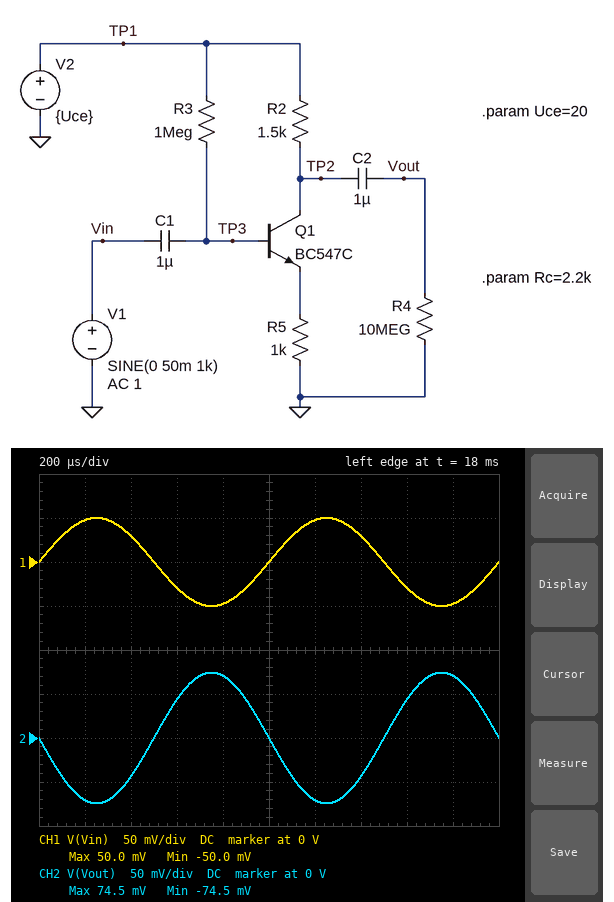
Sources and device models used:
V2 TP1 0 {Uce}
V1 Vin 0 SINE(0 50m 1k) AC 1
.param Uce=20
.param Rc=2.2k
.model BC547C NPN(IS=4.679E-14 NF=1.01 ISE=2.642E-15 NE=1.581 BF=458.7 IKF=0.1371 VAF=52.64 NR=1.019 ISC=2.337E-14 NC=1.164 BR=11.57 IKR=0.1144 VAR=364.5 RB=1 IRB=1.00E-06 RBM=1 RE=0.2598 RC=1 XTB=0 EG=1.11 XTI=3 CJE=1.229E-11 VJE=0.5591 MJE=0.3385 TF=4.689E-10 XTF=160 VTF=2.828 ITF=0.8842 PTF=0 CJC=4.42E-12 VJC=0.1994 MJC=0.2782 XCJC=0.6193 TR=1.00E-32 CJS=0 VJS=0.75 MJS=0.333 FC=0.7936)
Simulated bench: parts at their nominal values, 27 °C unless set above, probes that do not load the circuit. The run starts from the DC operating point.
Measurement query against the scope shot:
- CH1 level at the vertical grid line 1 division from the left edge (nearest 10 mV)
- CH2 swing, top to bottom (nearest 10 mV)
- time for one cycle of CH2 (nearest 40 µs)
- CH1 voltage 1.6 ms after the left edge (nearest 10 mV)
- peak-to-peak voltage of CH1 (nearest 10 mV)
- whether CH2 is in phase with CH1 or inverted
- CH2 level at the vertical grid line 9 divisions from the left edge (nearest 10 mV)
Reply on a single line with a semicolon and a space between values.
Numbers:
50 mV; 150 mV; 1.00 ms; -30 mV; 100 mV; inverted; 70 mV
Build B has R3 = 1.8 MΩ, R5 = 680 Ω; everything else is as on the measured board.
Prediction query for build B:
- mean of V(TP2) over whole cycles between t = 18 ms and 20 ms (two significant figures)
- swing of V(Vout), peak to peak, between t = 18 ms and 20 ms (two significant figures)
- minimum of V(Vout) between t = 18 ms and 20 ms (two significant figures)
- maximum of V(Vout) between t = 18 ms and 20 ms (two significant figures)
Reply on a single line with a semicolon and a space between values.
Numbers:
13 V; 220 mV; -110 mV; 110 mV
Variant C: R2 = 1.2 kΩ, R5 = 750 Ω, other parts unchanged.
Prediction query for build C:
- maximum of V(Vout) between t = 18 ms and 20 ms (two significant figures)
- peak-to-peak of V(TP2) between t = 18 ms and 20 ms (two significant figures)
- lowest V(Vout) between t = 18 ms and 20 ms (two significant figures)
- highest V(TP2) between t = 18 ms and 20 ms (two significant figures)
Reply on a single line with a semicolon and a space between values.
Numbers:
79 mV; 160 mV; -79 mV; 12 V
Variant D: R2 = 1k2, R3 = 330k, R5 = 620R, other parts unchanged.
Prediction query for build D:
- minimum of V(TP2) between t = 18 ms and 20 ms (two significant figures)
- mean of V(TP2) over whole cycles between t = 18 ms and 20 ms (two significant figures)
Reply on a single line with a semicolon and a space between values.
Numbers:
6.9 V; 7.0 V
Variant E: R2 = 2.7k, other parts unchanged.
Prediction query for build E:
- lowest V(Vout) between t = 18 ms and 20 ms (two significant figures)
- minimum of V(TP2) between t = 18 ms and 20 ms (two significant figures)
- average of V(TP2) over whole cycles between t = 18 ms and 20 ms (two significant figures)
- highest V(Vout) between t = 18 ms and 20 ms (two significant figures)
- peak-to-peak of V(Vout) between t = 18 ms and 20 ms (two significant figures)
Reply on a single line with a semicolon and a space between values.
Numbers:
-29 mV; 5.5 V; 5.6 V; 210 mV; 240 mV
